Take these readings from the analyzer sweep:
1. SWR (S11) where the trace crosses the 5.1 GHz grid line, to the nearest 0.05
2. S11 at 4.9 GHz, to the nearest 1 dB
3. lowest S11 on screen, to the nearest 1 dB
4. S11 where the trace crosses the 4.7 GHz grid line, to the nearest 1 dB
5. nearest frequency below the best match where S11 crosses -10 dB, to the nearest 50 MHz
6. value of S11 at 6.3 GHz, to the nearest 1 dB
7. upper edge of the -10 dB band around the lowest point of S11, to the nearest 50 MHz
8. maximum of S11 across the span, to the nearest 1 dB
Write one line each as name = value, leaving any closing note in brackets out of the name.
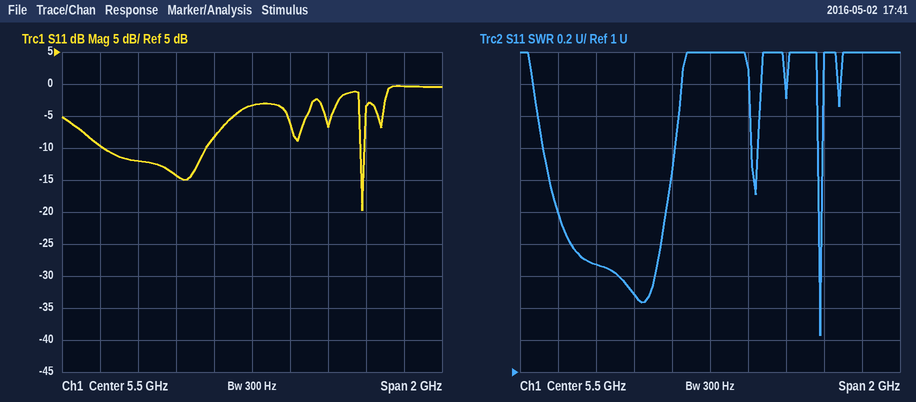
SWR (S11) where the trace crosses the 5.1 GHz grid line, to the nearest 0.05 = 1.50
S11 at 4.9 GHz, to the nearest 1 dB = -12 dB
lowest S11 on screen, to the nearest 1 dB = -20 dB
S11 where the trace crosses the 4.7 GHz grid line, to the nearest 1 dB = -10 dB
nearest frequency below the best match where S11 crosses -10 dB, to the nearest 50 MHz = 6.05 GHz
value of S11 at 6.3 GHz, to the nearest 1 dB = 0 dB
upper edge of the -10 dB band around the lowest point of S11, to the nearest 50 MHz = 6.10 GHz
maximum of S11 across the span, to the nearest 1 dB = 0 dB
